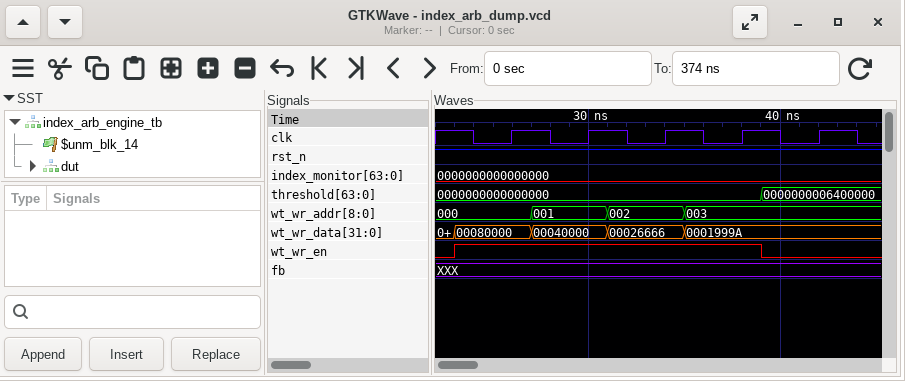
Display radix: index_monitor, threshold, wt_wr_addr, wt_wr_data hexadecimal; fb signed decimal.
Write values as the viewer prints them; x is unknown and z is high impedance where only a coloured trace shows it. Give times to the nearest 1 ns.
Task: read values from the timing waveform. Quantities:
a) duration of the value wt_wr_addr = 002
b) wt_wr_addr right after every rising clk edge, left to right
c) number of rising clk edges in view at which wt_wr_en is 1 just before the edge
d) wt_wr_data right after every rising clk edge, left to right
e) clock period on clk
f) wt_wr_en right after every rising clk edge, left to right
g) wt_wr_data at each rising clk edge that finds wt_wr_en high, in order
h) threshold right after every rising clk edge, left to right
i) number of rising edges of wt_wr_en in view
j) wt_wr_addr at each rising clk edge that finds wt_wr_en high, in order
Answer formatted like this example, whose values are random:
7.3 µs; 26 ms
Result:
4 ns; 000, 001, 002, 003, 003; 4; 00080000, 00040000, 00026666, 0001999A, 0001999A; 4 ns; 1 1 1 1 0; 00080000, 00040000, 00026666, 0001999A; 0000000000000000, 0000000000000000, 0000000000000000, 0000000000000000, 0000000006400000; 1; 000, 001, 002, 003
